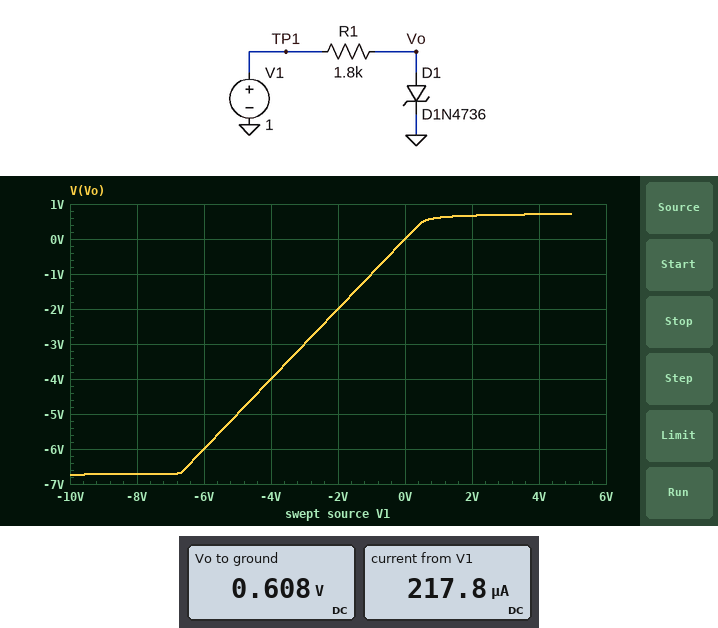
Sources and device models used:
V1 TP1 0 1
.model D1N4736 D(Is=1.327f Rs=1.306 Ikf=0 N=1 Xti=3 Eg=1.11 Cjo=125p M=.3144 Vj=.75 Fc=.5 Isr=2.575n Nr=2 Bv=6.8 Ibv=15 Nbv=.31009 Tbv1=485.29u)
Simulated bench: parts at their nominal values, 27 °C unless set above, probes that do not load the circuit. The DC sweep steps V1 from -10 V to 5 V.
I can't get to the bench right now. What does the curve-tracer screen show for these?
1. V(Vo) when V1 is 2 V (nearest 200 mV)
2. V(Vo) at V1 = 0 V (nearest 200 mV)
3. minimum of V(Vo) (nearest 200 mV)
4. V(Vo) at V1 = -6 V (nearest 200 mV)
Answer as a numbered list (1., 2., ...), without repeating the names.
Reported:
1. 600 mV
2. 0 V
3. -6.8 V
4. -6.0 V
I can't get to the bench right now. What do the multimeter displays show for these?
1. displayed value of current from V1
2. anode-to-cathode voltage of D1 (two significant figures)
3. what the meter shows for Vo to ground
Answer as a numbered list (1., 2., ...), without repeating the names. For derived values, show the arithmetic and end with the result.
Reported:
1. 217.8 µA
2. 608 mV = 610 mV
3. 0.608 V
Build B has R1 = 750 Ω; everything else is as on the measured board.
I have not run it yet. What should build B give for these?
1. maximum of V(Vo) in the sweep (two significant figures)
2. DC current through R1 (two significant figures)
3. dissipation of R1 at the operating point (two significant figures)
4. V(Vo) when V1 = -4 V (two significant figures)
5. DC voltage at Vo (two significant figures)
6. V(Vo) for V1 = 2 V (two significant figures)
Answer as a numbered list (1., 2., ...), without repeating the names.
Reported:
1. 750 mV
2. 470 µA
3. 170 µW
4. -4.0 V
5. 650 mV
6. 700 mV
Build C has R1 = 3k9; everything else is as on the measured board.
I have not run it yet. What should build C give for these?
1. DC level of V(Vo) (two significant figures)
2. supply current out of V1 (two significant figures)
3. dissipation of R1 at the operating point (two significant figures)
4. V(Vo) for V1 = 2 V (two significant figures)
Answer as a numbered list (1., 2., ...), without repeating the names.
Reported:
1. 570 mV
2. 110 µA
3. 47 µW
4. 630 mV
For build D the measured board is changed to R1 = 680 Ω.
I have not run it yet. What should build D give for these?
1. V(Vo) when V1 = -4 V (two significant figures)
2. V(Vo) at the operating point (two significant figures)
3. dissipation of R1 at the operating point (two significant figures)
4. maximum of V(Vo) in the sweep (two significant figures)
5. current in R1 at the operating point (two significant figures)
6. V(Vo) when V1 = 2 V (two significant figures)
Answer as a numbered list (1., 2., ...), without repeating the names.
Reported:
1. -4.0 V
2. 650 mV
3. 180 µW
4. 750 mV
5. 510 µA
6. 710 mV
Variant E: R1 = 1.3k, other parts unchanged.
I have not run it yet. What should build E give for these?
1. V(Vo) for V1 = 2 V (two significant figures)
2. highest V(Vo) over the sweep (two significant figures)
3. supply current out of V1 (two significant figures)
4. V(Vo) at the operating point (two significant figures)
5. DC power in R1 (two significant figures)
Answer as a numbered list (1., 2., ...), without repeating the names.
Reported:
1. 680 mV
2. 730 mV
3. 290 µA
4. 620 mV
5. 110 µW
